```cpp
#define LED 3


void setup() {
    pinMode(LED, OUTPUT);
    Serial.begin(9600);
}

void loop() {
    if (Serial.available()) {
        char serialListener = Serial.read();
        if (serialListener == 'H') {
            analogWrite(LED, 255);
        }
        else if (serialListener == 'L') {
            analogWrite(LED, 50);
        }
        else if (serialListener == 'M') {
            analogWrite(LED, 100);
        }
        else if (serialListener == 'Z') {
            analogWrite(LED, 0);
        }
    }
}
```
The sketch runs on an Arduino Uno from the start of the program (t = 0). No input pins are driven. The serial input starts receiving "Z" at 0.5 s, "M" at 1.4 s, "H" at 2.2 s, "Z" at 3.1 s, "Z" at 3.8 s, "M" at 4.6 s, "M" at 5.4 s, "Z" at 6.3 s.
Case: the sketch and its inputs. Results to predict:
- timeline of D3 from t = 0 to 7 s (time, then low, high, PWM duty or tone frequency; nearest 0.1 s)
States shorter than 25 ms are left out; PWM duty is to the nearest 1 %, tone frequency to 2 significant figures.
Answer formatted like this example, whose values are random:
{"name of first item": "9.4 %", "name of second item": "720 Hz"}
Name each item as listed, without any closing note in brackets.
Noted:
{"timeline of D3 from t = 0 to 7 s": "0 s low; 1.4 s PWM 39 %; 2.2 s high; 3.1 s low; 4.6 s PWM 39 %; 6.3 s low"}
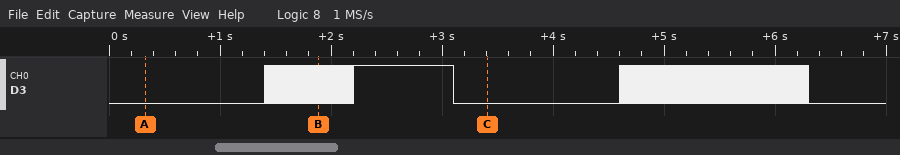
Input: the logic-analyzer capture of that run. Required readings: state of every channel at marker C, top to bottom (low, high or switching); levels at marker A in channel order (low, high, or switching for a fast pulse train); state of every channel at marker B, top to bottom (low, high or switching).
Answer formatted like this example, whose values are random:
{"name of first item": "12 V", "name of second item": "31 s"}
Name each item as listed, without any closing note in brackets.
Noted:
{"state of every channel at marker C, top to bottom": "D3 low", "levels at marker A in channel order": "D3 low", "state of every channel at marker B, top to bottom": "D3 switching"}
